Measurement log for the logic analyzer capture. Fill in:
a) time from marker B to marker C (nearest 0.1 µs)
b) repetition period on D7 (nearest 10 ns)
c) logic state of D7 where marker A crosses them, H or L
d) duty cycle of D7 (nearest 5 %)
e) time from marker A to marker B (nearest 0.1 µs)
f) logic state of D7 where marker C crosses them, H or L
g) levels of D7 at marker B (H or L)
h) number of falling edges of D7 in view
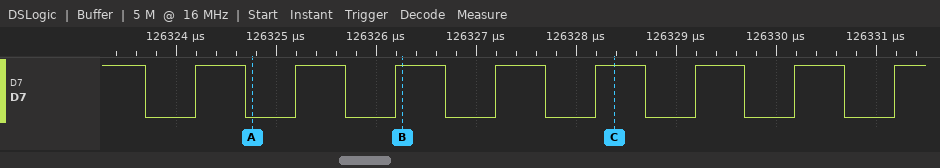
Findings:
2.1 µs
1000 ns
D7=L
50 %
1.5 µs
D7=H
D7=H
8
